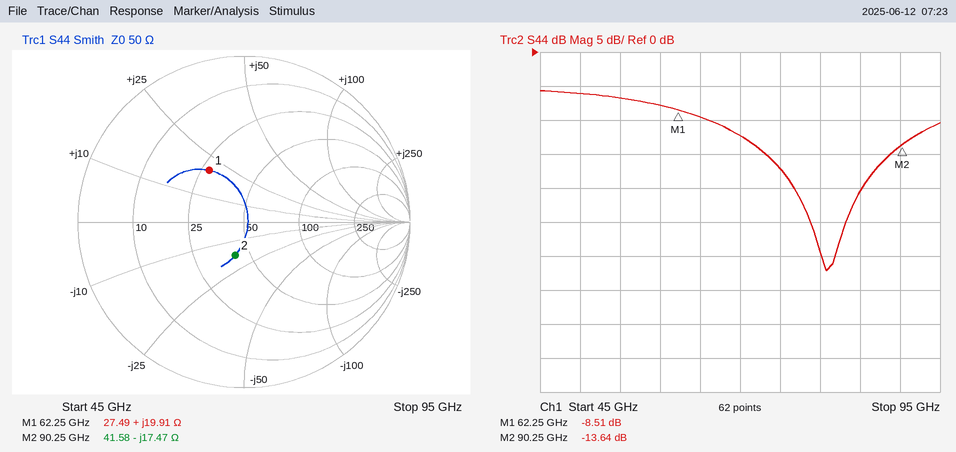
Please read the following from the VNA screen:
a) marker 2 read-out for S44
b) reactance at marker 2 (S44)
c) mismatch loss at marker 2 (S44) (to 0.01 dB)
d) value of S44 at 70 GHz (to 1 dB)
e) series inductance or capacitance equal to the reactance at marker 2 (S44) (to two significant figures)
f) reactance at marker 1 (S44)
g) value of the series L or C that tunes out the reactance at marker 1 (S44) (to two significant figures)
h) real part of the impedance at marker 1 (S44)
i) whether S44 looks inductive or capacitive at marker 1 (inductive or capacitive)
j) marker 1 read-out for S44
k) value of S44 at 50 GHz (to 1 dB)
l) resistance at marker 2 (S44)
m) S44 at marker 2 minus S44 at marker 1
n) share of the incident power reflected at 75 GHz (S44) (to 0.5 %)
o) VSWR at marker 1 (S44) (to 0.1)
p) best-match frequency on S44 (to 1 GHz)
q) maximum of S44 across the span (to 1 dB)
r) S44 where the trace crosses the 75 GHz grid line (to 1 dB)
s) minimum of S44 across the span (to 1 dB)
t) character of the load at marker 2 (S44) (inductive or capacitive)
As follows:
-13.64 dB
-17.47 Ω
0.19 dB
-12 dB
100 fF
+19.91 Ω
130 fF
27.49 Ω
inductive
-8.51 dB
-6 dB
41.58 Ω
-5.13 dB
2.0 %
2.2
81 GHz
-6 dB
-17 dB
-32 dB
capacitive
